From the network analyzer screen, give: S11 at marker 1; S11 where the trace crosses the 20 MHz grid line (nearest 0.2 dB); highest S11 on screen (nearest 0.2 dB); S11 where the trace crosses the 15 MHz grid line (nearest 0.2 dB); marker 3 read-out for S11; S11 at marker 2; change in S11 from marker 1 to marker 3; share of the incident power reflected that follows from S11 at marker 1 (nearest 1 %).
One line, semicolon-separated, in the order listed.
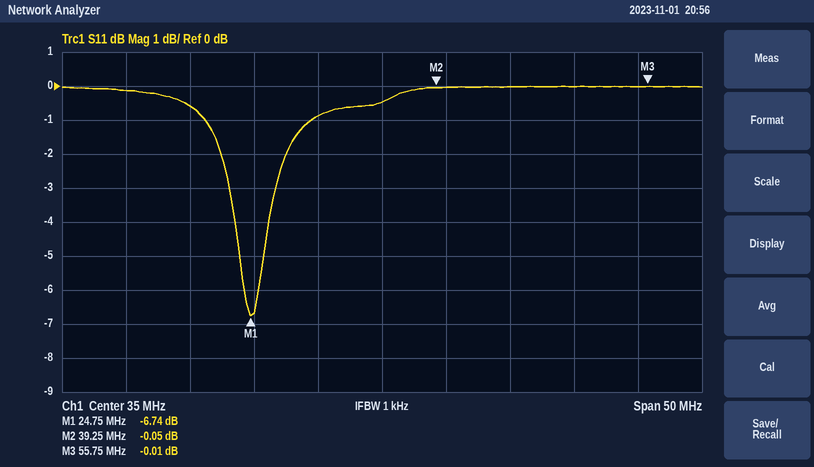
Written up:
-6.74 dB; -0.6 dB; 0.0 dB; -0.2 dB; -0.01 dB; -0.05 dB; 6.73 dB; 21 %
